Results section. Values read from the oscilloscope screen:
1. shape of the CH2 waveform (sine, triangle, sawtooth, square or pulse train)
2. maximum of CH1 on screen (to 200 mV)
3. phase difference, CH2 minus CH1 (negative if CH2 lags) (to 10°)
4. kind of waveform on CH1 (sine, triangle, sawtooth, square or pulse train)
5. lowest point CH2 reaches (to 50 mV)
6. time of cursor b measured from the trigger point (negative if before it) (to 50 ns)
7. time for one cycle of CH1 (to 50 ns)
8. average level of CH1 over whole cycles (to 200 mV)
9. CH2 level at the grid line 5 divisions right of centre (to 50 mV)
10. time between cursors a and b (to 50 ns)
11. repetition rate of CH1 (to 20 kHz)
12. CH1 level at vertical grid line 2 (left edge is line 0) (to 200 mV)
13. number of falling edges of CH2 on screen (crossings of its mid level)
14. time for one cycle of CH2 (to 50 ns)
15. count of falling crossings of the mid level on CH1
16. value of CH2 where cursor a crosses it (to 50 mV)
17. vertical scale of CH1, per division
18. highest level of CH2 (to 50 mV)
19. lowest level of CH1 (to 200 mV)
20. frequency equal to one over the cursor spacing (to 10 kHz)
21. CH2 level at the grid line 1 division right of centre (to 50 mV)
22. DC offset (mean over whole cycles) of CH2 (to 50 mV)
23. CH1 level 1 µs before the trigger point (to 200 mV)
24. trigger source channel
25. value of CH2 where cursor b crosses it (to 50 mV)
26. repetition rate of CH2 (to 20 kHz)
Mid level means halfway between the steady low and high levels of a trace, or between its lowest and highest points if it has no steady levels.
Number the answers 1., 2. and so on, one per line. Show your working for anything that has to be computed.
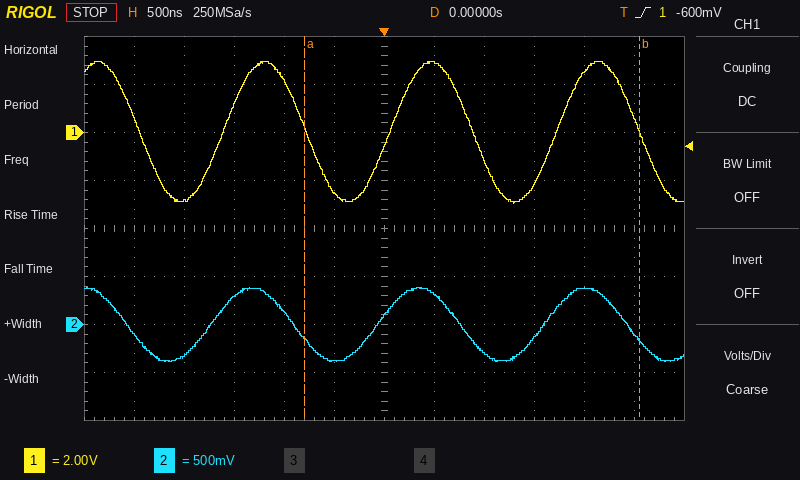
1. sine
2. 3.0 V
3. +30°
4. sine
5. -400 mV
6. +2.55 µs
7. 1.65 µs
8. (3.0 V + (-3.0 V)) / 2 ≈ 0.0 V
9. -100 mV
10. 3.35 µs
11. 1 / 1.65 µs ≈ 606 kHz, so 600 kHz to the nearest 20 kHz
12. -2.8 V
13. 4
14. 1.65 µs
15. 4
16. -150 mV
17. 2 V
18. 400 mV
19. -3.0 V
20. 1 / 3.35 µs ≈ 300 kHz
21. 300 mV
22. (400 mV + (-400 mV)) / 2 ≈ 0 mV
23. 2.2 V
24. CH1
25. -150 mV
26. 1 / 1.65 µs ≈ 606 kHz, so 600 kHz to the nearest 20 kHz
